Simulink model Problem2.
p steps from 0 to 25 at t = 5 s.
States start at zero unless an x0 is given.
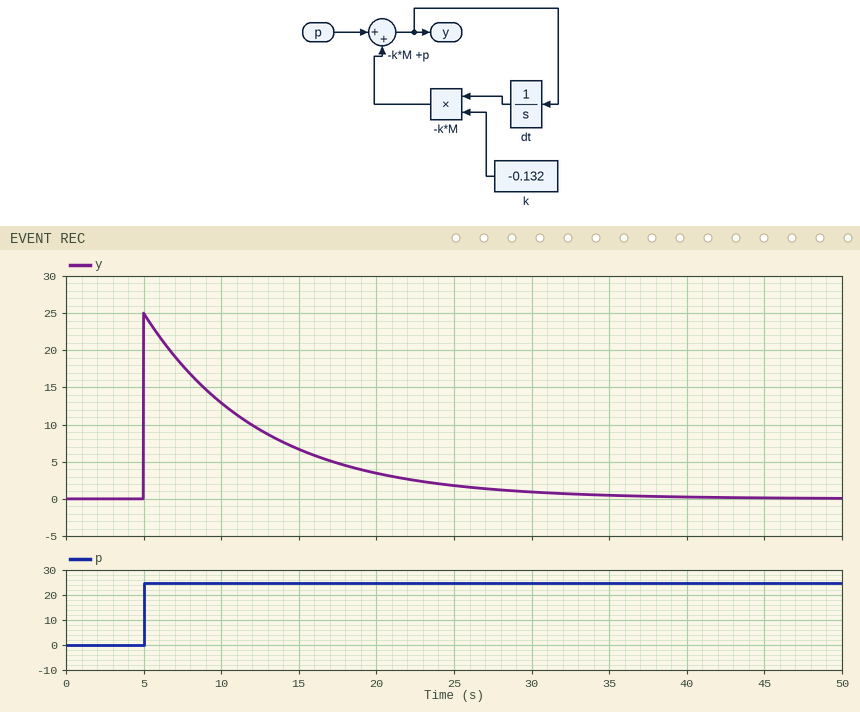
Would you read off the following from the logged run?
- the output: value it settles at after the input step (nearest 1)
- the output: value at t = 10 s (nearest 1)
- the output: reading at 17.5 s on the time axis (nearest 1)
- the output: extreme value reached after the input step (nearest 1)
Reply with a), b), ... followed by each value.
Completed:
a) 0
b) 13
c) 5
d) 25
